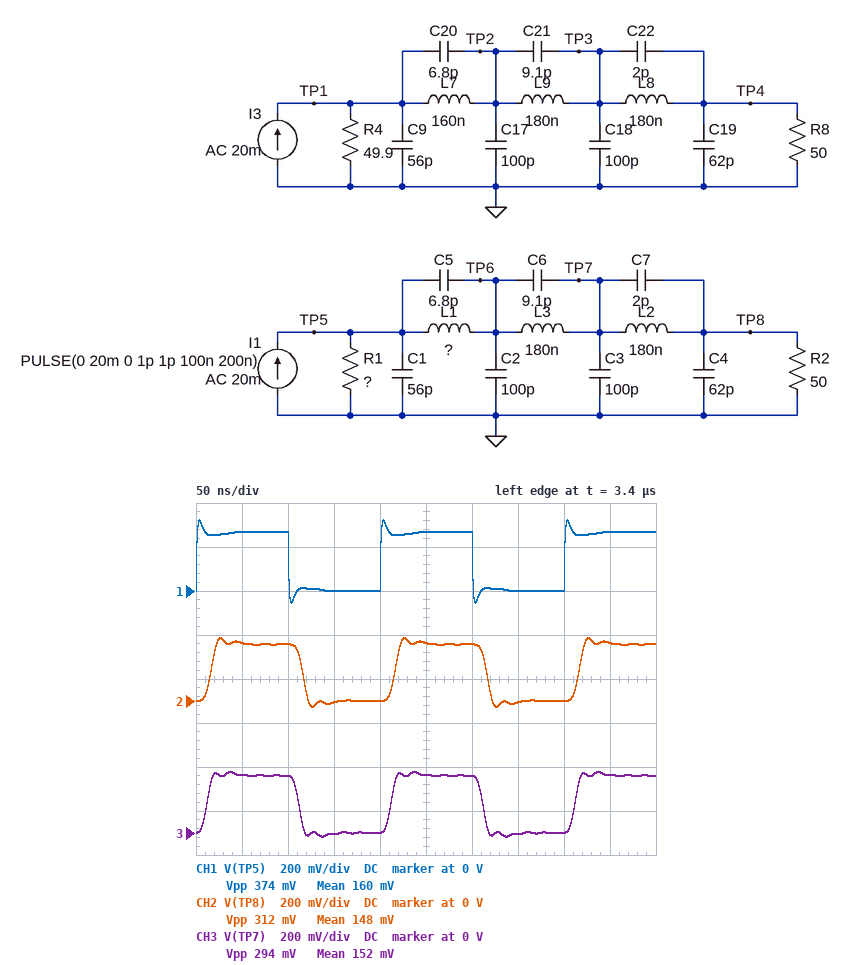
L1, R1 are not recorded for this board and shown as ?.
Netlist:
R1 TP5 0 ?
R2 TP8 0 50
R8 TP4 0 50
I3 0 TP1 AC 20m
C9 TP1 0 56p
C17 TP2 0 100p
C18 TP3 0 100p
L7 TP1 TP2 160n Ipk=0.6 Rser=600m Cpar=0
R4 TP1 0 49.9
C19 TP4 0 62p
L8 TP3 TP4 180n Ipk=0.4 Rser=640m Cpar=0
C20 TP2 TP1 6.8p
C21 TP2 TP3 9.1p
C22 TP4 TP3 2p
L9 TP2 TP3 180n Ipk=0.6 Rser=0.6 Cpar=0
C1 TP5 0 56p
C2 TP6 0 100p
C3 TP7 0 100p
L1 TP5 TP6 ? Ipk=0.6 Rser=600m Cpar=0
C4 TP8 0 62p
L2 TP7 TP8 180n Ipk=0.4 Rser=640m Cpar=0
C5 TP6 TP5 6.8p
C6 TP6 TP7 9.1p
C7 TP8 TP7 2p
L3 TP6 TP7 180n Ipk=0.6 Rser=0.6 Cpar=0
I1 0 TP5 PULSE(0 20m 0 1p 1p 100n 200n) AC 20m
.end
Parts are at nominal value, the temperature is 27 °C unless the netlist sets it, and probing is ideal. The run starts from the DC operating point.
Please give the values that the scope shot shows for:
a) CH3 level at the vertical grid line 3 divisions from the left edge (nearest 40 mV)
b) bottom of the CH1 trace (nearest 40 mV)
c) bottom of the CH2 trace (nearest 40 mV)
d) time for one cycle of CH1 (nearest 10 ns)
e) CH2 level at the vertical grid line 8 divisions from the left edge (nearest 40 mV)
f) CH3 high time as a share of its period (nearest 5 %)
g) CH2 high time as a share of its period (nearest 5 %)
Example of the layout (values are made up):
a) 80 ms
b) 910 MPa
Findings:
a) 0 V
b) -40 mV
c) -40 mV
d) 200 ns
e) 0 V
f) 50 %
g) 50 %
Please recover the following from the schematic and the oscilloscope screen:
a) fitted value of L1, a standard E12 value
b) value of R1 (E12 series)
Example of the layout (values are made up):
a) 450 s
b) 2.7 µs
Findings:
a) 330 nH
b) 18 Ω
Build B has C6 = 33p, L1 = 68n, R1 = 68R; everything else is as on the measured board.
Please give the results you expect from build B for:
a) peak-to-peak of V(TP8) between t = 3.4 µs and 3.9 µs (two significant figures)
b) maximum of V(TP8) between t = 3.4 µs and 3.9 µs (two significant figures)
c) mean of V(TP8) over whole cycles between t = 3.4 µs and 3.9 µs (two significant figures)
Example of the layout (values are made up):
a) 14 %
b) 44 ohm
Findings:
a) 690 mV
b) 630 mV
c) 280 mV
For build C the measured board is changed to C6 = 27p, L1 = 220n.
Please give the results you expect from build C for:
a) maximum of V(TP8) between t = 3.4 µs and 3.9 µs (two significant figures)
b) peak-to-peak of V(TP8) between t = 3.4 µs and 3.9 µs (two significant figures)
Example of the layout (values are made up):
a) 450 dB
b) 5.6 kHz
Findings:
a) 310 mV
b) 360 mV
